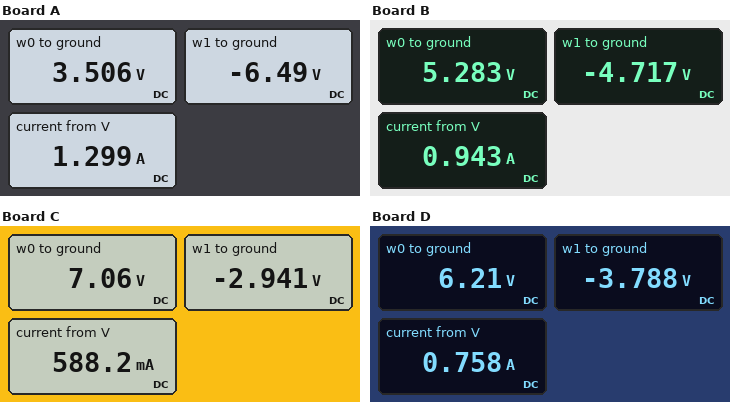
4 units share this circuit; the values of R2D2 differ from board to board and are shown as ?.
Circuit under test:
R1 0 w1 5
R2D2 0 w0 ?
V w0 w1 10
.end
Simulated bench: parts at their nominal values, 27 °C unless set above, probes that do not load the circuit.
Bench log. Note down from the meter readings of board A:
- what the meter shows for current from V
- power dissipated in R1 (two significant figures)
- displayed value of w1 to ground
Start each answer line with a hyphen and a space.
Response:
- 1.299 A
- 8.4 W
- -6.49 V
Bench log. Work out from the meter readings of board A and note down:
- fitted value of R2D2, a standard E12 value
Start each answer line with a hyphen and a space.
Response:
- 2.7 Ω
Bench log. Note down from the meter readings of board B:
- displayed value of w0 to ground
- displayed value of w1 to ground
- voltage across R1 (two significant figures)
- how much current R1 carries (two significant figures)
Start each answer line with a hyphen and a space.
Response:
- 5.283 V
- -4.717 V
- 4.7 V
- 940 mA
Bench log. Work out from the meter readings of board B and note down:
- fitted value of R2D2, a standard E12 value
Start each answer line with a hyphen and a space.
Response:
- 5.6 Ω
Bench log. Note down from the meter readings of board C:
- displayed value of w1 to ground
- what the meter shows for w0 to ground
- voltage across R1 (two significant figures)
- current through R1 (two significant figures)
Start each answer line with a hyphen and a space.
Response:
- -2.941 V
- 7.06 V
- 2.9 V
- 590 mA
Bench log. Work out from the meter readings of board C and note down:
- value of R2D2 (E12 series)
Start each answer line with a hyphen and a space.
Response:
- 12 Ω
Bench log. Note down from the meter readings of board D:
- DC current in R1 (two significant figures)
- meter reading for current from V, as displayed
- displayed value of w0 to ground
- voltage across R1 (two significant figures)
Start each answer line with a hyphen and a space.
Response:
- 760 mA
- 0.758 A
- 6.21 V
- 3.8 V
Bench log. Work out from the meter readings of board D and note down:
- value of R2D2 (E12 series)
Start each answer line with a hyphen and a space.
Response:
- 8.2 Ω
